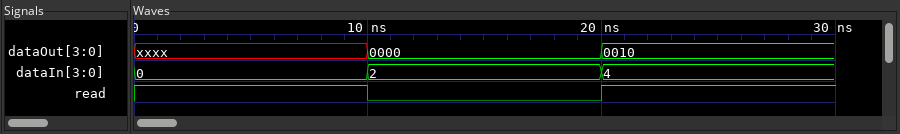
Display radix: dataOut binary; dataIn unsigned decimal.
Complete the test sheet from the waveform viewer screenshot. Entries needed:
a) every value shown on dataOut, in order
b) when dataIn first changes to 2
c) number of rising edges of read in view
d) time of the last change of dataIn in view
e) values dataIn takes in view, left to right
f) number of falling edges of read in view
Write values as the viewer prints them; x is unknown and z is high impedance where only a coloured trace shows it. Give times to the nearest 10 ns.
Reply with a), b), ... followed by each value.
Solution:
a) xxxx, 0000, 0010
b) 10 ns
c) 1
d) 20 ns
e) 0, 2, 4
f) 1
